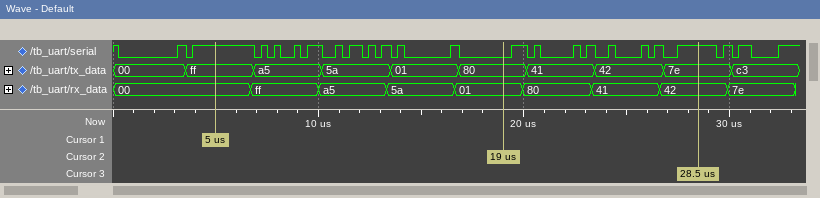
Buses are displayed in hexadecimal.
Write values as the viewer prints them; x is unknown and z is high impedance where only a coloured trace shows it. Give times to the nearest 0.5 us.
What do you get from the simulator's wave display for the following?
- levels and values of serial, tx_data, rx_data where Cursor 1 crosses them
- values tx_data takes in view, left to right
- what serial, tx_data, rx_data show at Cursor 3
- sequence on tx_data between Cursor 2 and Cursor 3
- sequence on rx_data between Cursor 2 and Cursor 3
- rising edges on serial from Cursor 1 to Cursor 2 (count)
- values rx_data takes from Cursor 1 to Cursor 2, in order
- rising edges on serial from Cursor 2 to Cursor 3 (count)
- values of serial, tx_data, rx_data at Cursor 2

serial=1, tx_data=ff, rx_data=00
00, ff, a5, 5a, 01, 80, 41, 42, 7e, c3
serial=1, tx_data=7e, rx_data=42
80, 41, 42, 7e
01, 80, 41, 42
10
00, ff, a5, 5a, 01
8
serial=0, tx_data=80, rx_data=01
